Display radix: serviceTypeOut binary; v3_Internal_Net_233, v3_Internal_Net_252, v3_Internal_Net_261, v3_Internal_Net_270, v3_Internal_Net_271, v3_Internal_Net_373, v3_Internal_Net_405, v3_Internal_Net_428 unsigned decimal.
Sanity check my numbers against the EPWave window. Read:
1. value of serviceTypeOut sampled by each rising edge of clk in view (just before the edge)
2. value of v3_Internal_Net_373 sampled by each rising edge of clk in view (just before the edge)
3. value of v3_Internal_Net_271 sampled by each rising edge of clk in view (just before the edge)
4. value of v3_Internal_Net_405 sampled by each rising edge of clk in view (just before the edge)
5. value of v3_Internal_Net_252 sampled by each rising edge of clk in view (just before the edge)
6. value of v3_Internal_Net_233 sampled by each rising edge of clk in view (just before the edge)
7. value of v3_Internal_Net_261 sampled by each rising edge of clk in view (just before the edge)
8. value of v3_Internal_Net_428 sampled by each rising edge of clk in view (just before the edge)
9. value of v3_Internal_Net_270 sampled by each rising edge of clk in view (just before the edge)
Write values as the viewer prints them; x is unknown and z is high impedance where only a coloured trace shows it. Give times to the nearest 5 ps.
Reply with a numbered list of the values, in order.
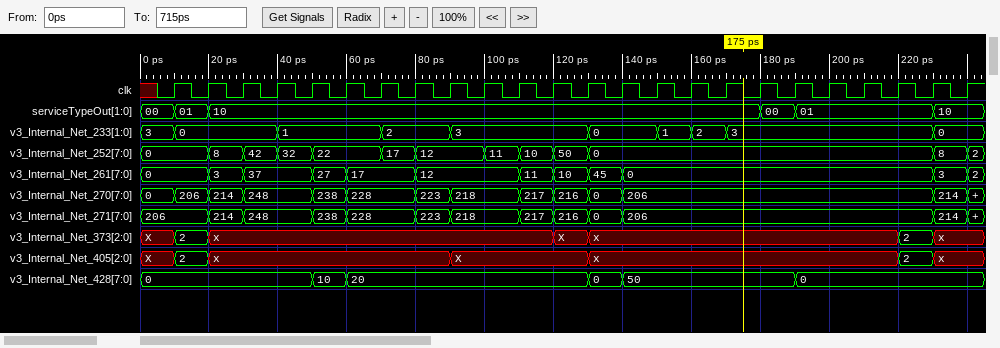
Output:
1. 00, 01, 10, 10, 10, 10, 10, 10, 10, 10, 10, 10, 10, 10, 10, 10, 10, 10, 00, 01, 01, 01, 01, 10
2. X, 2, x, x, x, x, x, x, x, x, x, x, X, x, x, x, x, x, x, x, x, x, 2, x
3. 206, 206, 214, 248, 248, 238, 228, 228, 223, 218, 218, 217, 216, 0, 206, 206, 206, 206, 206, 206, 206, 206, 206, 214
4. X, 2, x, x, x, x, x, x, x, X, X, X, X, x, x, x, x, x, x, x, x, x, 2, x
5. 0, 0, 8, 42, 32, 22, 22, 17, 12, 12, 11, 10, 50, 0, 0, 0, 0, 0, 0, 0, 0, 0, 0, 8
6. 3, 0, 0, 0, 1, 1, 1, 2, 2, 3, 3, 3, 3, 0, 0, 1, 2, 3, 3, 3, 3, 3, 3, 0
7. 0, 0, 3, 37, 37, 27, 17, 17, 12, 12, 12, 11, 10, 45, 0, 0, 0, 0, 0, 0, 0, 0, 0, 3
8. 0, 0, 0, 0, 0, 10, 20, 20, 20, 20, 20, 20, 20, 0, 50, 50, 50, 50, 50, 0, 0, 0, 0, 0
9. 0, 206, 214, 248, 248, 238, 228, 228, 223, 218, 218, 217, 216, 0, 206, 206, 206, 206, 206, 206, 206, 206, 206, 214
